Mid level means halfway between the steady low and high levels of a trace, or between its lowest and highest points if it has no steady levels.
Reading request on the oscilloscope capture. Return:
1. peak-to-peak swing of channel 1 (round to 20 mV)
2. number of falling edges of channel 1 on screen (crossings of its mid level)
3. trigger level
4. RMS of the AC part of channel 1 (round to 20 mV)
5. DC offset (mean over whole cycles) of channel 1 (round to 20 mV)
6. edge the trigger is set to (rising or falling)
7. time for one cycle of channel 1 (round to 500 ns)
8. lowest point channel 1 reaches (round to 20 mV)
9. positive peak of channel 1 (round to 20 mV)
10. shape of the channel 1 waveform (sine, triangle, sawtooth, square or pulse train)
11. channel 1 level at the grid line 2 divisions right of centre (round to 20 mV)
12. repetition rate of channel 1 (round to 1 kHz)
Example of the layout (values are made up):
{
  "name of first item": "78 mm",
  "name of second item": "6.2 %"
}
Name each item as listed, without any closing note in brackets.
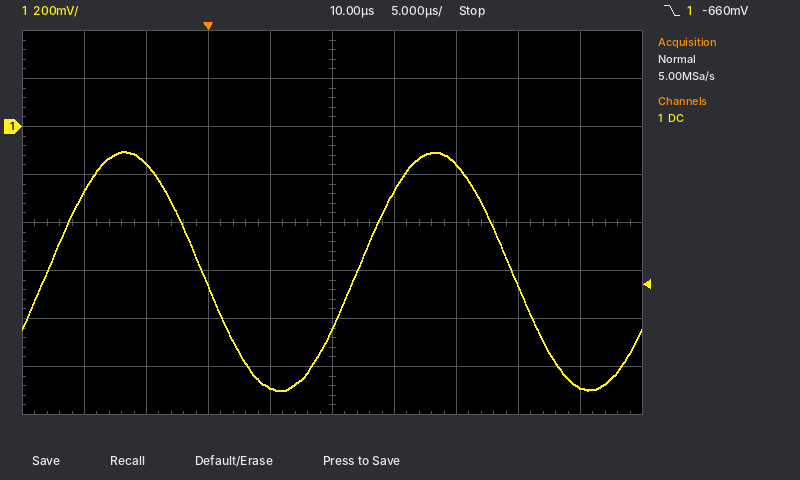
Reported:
{
  "peak-to-peak swing of channel 1": "1.00 V",
  "number of falling edges of channel 1 on screen": "2",
  "trigger level": "-660 mV",
  "RMS of the AC part of channel 1": "360 mV",
  "DC offset (mean over whole cycles) of channel 1": "-600 mV",
  "edge the trigger is set to": "falling",
  "time for one cycle of channel 1": "25.0 µs",
  "lowest point channel 1 reaches": "-1.10 V",
  "positive peak of channel 1": "-100 mV",
  "shape of the channel 1 waveform": "sine",
  "channel 1 level at the grid line 2 divisions right of centre": "-160 mV",
  "repetition rate of channel 1": "40 kHz"
}
